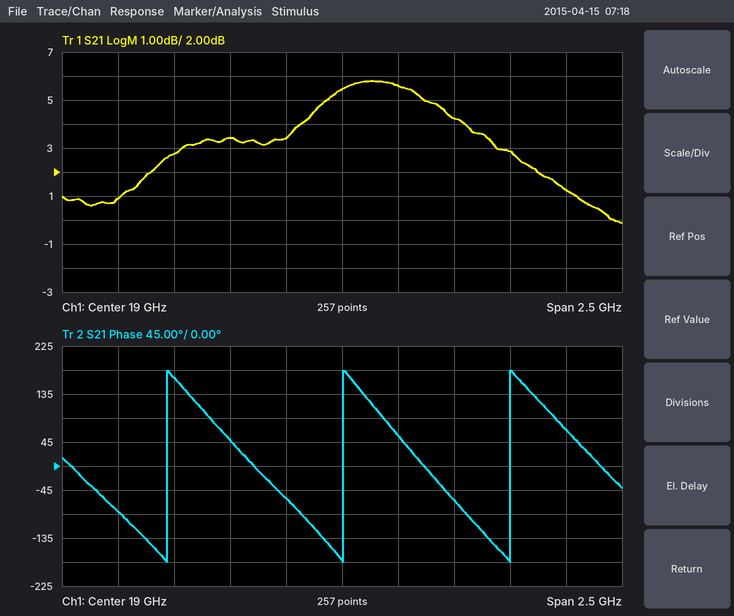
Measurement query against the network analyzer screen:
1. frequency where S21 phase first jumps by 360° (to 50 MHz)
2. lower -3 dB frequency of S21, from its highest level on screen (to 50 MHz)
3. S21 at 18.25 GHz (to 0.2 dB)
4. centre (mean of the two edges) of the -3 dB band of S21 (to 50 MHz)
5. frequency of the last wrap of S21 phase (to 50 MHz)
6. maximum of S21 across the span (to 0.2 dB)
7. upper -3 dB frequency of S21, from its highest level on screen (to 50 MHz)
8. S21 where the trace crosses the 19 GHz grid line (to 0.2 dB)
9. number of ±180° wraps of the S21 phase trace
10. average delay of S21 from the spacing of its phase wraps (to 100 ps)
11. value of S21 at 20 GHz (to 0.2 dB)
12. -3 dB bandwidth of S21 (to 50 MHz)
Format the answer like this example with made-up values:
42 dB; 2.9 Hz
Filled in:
18.20 GHz; 18.25 GHz; 2.8 dB; 19.00 GHz; 19.75 GHz; 5.8 dB; 19.75 GHz; 5.4 dB; 3; 1.3 ns; 1.2 dB; 1.50 GHz
